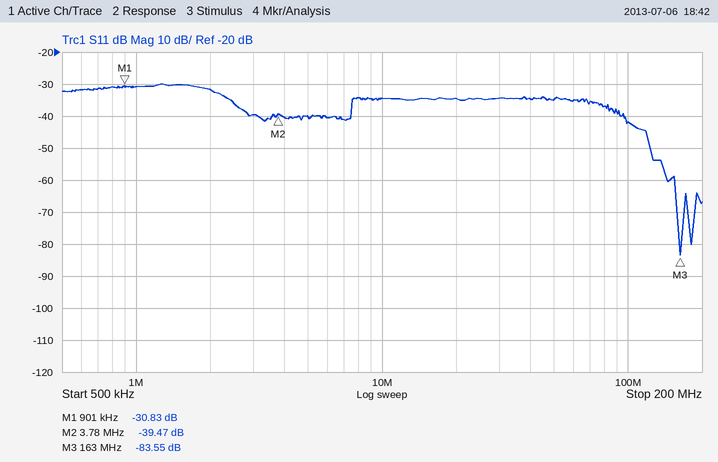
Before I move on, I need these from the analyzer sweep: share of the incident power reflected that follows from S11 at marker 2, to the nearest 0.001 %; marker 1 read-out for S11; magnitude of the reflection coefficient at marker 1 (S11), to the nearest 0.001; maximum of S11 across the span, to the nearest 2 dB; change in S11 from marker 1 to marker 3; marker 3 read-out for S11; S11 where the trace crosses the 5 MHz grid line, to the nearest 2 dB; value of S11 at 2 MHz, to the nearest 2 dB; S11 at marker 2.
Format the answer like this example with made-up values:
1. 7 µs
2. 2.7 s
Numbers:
1. 0.011 %
2. -30.83 dB
3. 0.029
4. -30 dB
5. -52.72 dB
6. -83.55 dB
7. -40 dB
8. -32 dB
9. -39.47 dB
